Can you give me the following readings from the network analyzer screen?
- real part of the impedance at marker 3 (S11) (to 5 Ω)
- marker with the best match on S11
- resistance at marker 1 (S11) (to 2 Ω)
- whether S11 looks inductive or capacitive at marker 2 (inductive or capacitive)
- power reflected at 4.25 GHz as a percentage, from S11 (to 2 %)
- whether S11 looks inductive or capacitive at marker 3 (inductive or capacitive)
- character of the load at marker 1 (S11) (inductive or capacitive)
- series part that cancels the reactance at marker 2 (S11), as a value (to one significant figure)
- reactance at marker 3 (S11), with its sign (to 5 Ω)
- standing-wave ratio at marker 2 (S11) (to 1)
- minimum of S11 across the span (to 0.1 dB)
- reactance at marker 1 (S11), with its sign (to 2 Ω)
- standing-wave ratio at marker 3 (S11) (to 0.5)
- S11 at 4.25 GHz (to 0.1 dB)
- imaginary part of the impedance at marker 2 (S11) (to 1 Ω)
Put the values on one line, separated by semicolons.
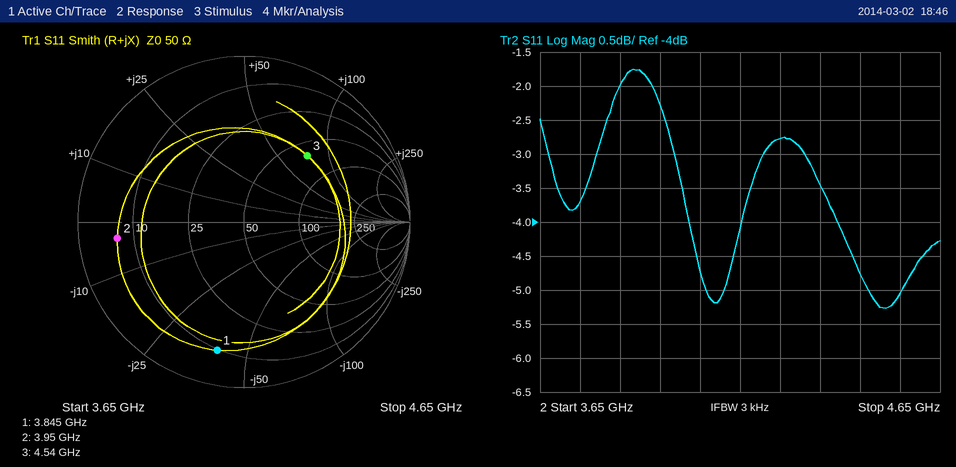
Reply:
65 Ω; marker 3; 10 Ω; capacitive; 52 %; inductive; capacitive; 100 pH; +75 Ω; 8; -5.3 dB; -40 Ω; 3.5; -2.8 dB; -3 Ω
